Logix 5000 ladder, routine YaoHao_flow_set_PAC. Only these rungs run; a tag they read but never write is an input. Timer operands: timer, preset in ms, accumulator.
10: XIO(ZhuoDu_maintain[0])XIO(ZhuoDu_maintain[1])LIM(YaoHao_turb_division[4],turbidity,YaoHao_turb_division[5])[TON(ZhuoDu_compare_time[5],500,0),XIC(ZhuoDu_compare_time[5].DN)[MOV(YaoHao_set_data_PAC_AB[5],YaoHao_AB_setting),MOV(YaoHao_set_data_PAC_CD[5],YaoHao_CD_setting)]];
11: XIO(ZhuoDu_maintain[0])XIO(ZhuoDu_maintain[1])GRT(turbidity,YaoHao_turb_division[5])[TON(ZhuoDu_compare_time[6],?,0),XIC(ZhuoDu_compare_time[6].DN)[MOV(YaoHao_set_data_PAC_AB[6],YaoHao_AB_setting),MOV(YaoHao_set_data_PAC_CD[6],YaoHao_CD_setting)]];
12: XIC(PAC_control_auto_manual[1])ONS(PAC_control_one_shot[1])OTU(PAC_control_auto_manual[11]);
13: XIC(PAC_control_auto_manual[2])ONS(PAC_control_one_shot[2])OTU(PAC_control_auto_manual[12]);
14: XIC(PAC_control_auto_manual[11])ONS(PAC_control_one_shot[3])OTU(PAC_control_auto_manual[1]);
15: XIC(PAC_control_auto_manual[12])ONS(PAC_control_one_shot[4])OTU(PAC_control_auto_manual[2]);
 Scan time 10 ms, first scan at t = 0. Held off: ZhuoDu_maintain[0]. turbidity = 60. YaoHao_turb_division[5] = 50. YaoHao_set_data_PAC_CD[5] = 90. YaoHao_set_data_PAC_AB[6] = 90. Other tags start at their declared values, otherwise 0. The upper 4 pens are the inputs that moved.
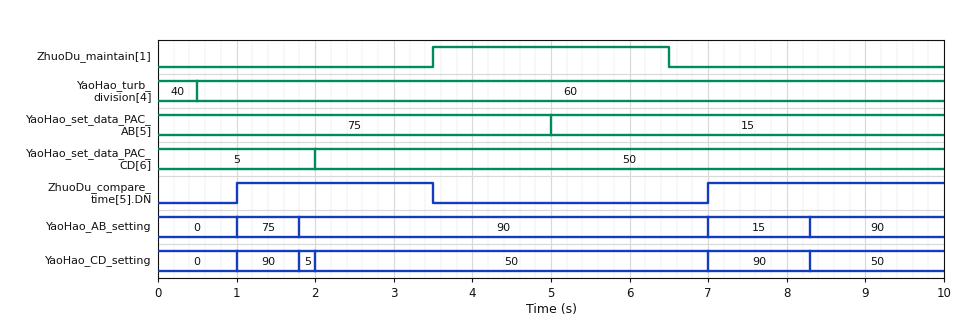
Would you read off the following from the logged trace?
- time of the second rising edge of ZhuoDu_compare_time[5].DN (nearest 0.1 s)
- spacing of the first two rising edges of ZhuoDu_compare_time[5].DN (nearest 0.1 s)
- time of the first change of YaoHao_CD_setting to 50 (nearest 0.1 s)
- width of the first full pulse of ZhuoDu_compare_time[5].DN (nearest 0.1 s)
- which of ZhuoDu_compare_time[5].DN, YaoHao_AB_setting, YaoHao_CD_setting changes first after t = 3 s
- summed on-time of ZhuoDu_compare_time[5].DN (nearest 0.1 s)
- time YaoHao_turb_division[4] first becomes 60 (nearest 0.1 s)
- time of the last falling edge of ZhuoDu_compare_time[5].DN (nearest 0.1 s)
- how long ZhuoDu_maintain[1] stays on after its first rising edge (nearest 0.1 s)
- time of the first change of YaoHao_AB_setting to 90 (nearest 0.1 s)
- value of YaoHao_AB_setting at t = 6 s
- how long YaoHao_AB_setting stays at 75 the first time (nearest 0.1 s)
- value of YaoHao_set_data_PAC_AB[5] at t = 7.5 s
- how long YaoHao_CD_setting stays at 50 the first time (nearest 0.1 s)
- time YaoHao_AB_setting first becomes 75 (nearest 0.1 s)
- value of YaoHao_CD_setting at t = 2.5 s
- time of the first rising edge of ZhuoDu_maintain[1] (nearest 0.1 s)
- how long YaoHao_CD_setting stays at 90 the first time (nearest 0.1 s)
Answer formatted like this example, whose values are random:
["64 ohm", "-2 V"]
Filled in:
["7.0 s", "6.0 s", "2.0 s", "2.5 s", "ZhuoDu_compare_time[5].DN", "5.5 s", "0.5 s", "3.5 s", "3.0 s", "1.8 s", "90", "0.8 s", "15", "5.0 s", "1.0 s", "50", "3.5 s", "0.8 s"]
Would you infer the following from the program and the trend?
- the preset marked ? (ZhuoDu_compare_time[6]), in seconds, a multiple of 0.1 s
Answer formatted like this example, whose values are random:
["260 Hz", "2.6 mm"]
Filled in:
["1.8 s"]
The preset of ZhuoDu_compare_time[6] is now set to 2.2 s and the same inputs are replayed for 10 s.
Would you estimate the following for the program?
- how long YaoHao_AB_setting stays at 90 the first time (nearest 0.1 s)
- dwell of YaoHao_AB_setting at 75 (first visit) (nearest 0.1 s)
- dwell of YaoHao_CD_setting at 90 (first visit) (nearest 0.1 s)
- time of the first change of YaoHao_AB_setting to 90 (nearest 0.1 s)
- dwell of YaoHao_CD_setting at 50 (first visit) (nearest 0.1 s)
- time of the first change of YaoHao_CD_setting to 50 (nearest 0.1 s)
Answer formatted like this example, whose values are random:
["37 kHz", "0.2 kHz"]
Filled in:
["4.8 s", "1.2 s", "1.2 s", "2.2 s", "4.8 s", "2.2 s"]
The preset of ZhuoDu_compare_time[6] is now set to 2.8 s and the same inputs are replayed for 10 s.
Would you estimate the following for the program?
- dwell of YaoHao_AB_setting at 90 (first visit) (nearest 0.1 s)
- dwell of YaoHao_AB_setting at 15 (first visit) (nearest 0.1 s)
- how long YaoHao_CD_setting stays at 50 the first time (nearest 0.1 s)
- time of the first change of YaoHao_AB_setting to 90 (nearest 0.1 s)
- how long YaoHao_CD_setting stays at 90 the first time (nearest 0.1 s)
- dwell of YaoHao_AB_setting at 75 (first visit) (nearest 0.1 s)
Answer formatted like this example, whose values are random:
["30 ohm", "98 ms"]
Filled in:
["4.2 s", "2.3 s", "4.2 s", "2.8 s", "1.8 s", "1.8 s"]
